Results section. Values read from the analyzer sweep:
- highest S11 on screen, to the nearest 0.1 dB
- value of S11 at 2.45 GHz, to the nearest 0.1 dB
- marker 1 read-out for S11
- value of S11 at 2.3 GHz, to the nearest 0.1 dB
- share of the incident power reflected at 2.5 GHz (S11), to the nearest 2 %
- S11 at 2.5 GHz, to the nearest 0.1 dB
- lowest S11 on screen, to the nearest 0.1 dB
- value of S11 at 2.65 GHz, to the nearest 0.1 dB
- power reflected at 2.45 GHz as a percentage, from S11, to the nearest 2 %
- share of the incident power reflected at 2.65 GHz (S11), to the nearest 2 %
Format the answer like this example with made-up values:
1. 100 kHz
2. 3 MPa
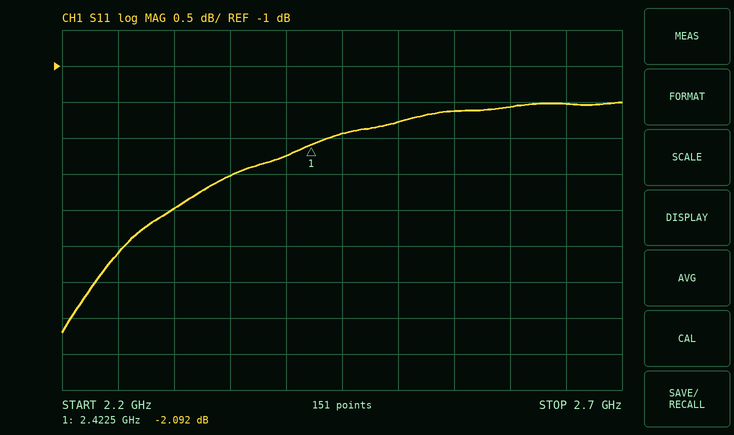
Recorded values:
1. -1.5 dB
2. -1.9 dB
3. -2.092 dB
4. -3.0 dB
5. 66 %
6. -1.8 dB
7. -4.7 dB
8. -1.5 dB
9. 64 %
10. 70 %
